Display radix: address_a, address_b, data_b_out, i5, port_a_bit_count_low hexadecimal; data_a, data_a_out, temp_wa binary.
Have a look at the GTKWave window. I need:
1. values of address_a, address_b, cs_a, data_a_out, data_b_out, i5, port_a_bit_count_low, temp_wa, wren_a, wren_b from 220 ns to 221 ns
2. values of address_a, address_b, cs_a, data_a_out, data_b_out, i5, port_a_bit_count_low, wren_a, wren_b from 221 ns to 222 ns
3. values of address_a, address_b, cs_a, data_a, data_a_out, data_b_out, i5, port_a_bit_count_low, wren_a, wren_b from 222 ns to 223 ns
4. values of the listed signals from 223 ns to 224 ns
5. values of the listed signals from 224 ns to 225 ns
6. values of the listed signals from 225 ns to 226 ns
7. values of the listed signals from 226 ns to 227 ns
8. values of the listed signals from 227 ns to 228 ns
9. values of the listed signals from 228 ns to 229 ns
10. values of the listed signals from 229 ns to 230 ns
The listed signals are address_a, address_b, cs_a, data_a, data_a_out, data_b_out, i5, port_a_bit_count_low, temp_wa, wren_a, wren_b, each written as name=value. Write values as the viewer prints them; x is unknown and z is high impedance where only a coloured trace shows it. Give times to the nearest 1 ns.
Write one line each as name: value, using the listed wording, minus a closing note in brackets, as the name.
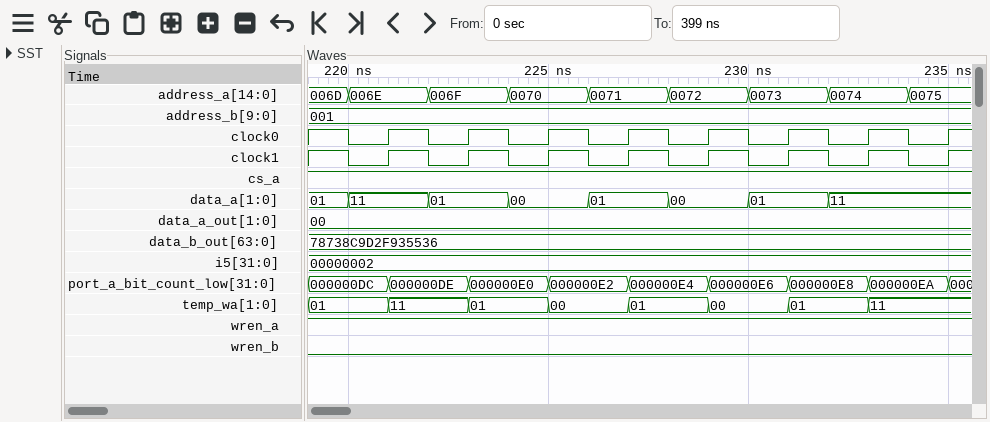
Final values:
values of address_a, address_b, cs_a, data_a_out, data_b_out, i5, port_a_bit_count_low, temp_wa, wren_a, wren_b from 220 ns to 221 ns: address_a=006E, address_b=001, cs_a=1, data_a_out=00, data_b_out=78738C9D2F935536, i5=00000002, port_a_bit_count_low=000000DC, temp_wa=01, wren_a=1, wren_b=0
values of address_a, address_b, cs_a, data_a_out, data_b_out, i5, port_a_bit_count_low, wren_a, wren_b from 221 ns to 222 ns: address_a=006E, address_b=001, cs_a=1, data_a_out=00, data_b_out=78738C9D2F935536, i5=00000002, port_a_bit_count_low=000000DE, wren_a=1, wren_b=0
values of address_a, address_b, cs_a, data_a, data_a_out, data_b_out, i5, port_a_bit_count_low, wren_a, wren_b from 222 ns to 223 ns: address_a=006F, address_b=001, cs_a=1, data_a=01, data_a_out=00, data_b_out=78738C9D2F935536, i5=00000002, port_a_bit_count_low=000000DE, wren_a=1, wren_b=0
values of the listed signals from 223 ns to 224 ns: address_a=006F, address_b=001, cs_a=1, data_a=01, data_a_out=00, data_b_out=78738C9D2F935536, i5=00000002, port_a_bit_count_low=000000E0, temp_wa=01, wren_a=1, wren_b=0
values of the listed signals from 224 ns to 225 ns: address_a=0070, address_b=001, cs_a=1, data_a=00, data_a_out=00, data_b_out=78738C9D2F935536, i5=00000002, port_a_bit_count_low=000000E0, temp_wa=01, wren_a=1, wren_b=0
values of the listed signals from 225 ns to 226 ns: address_a=0070, address_b=001, cs_a=1, data_a=00, data_a_out=00, data_b_out=78738C9D2F935536, i5=00000002, port_a_bit_count_low=000000E2, temp_wa=00, wren_a=1, wren_b=0
values of the listed signals from 226 ns to 227 ns: address_a=0071, address_b=001, cs_a=1, data_a=01, data_a_out=00, data_b_out=78738C9D2F935536, i5=00000002, port_a_bit_count_low=000000E2, temp_wa=00, wren_a=1, wren_b=0
values of the listed signals from 227 ns to 228 ns: address_a=0071, address_b=001, cs_a=1, data_a=01, data_a_out=00, data_b_out=78738C9D2F935536, i5=00000002, port_a_bit_count_low=000000E4, temp_wa=01, wren_a=1, wren_b=0
values of the listed signals from 228 ns to 229 ns: address_a=0072, address_b=001, cs_a=1, data_a=00, data_a_out=00, data_b_out=78738C9D2F935536, i5=00000002, port_a_bit_count_low=000000E4, temp_wa=01, wren_a=1, wren_b=0
values of the listed signals from 229 ns to 230 ns: address_a=0072, address_b=001, cs_a=1, data_a=00, data_a_out=00, data_b_out=78738C9D2F935536, i5=00000002, port_a_bit_count_low=000000E6, temp_wa=00, wren_a=1, wren_b=0
